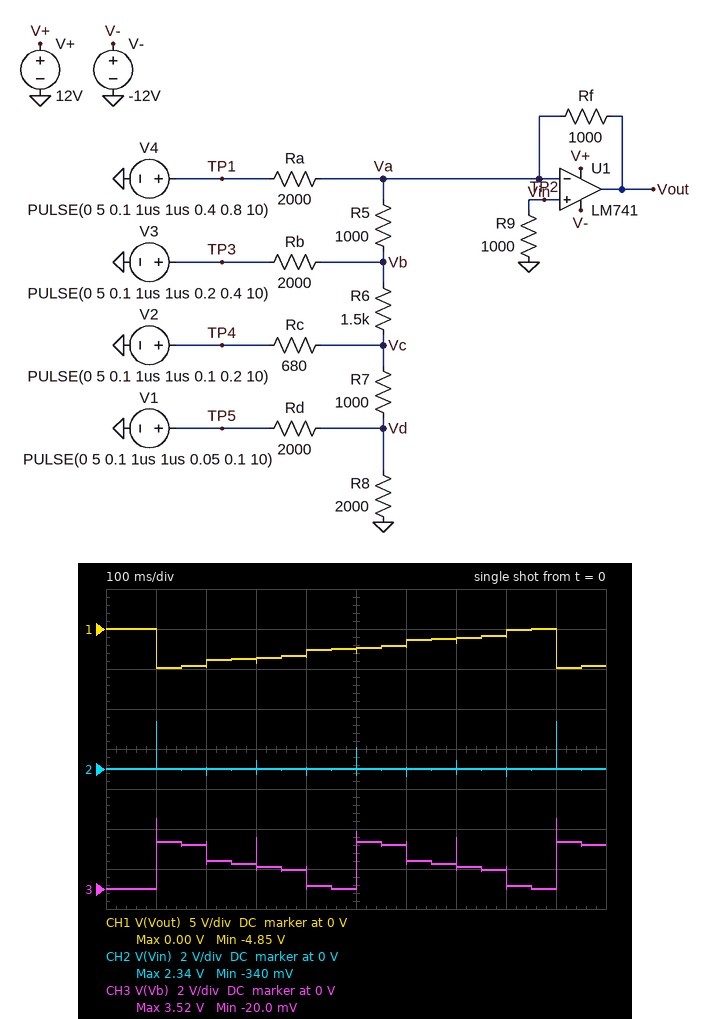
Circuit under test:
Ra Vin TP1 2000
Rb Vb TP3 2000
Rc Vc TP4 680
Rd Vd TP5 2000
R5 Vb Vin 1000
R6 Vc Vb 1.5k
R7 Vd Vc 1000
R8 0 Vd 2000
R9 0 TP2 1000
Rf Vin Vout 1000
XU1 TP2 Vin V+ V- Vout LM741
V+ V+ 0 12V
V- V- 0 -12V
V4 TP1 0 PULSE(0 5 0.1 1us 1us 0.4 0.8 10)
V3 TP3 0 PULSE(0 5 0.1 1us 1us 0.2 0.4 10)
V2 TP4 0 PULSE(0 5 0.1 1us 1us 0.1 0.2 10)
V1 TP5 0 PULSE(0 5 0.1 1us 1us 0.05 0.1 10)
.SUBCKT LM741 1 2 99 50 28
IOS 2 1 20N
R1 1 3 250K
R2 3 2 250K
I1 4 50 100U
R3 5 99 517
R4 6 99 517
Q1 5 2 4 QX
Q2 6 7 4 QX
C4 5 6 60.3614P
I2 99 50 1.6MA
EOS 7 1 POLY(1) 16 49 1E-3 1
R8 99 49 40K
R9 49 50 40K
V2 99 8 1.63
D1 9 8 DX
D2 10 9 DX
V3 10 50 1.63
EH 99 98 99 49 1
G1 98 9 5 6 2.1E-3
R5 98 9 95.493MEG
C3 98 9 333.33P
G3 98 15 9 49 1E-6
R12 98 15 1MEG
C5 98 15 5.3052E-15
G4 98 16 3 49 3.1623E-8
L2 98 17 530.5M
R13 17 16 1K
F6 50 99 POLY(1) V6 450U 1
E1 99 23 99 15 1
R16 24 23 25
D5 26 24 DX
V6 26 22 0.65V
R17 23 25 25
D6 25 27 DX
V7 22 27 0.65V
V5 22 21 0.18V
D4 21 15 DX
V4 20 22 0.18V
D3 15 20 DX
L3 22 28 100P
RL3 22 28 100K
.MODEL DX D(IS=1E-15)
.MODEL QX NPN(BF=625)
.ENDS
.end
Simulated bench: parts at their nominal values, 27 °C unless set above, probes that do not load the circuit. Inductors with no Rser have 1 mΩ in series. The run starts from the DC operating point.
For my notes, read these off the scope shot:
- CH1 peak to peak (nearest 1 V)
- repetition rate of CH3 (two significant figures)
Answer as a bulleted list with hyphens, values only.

- 5 V
- 2.5 Hz
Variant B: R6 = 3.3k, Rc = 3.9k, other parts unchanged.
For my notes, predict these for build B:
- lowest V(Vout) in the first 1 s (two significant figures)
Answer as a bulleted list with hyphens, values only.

- -4.4 V
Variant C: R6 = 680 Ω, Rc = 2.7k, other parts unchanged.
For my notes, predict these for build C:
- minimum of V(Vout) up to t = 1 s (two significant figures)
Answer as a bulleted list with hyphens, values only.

- -4.7 V
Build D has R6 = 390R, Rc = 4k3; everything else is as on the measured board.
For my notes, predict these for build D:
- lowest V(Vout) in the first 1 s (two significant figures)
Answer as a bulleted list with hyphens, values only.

- -4.6 V
